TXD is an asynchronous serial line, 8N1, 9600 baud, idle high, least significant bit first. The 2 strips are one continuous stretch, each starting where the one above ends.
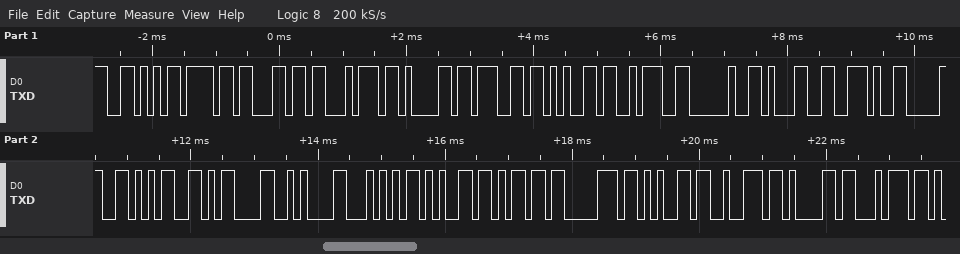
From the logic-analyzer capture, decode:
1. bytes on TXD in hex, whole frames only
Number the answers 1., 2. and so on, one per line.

1. 56 6F 6C 74 61 67 65 3A 20 31 2E 30 35 0D 0A 54 65 6D 70 65 72 61 74
